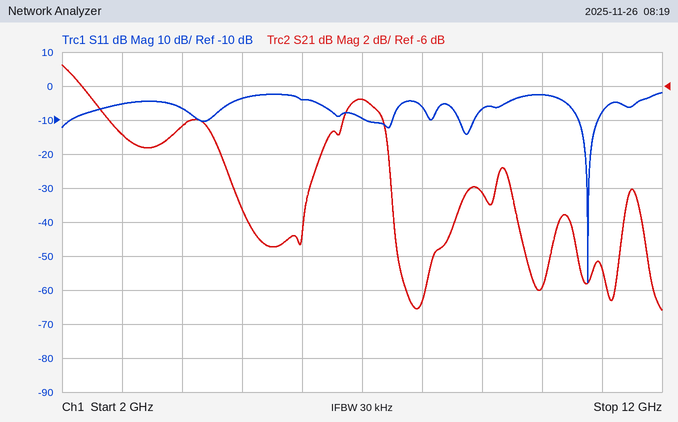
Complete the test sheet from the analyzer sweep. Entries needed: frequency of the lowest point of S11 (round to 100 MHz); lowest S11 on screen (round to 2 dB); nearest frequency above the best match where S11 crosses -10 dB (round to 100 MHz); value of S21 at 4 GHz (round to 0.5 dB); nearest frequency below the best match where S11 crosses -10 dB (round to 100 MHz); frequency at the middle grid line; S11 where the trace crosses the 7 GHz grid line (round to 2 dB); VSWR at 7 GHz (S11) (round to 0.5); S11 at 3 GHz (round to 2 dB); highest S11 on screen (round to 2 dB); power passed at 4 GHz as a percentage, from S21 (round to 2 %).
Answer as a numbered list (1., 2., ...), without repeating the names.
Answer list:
1. 10.8 GHz
2. -58 dB
3. 10.9 GHz
4. -8.5 dB
5. 10.6 GHz
6. 7 GHz
7. -10 dB
8. 2.0
9. -6 dB
10. -2 dB
11. 14 %
